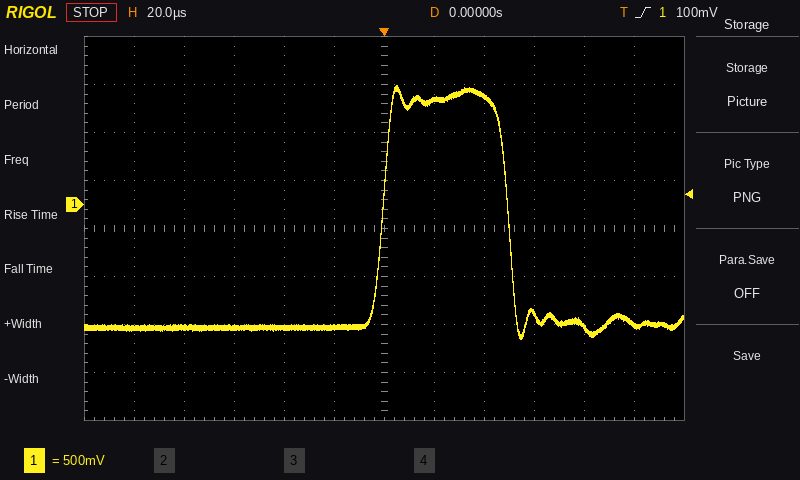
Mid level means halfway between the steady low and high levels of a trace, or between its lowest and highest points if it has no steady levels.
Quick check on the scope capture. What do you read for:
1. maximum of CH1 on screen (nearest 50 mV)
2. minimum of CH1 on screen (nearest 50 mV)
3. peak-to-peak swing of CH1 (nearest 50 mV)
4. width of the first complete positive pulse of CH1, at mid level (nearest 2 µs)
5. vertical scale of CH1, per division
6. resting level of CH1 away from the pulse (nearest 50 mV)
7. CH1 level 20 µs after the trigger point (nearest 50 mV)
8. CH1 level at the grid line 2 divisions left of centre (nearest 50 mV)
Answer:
1.25 V
-1.40 V
2.65 V
50 µs
500 mV
-1.30 V
1.10 V
-1.30 V
